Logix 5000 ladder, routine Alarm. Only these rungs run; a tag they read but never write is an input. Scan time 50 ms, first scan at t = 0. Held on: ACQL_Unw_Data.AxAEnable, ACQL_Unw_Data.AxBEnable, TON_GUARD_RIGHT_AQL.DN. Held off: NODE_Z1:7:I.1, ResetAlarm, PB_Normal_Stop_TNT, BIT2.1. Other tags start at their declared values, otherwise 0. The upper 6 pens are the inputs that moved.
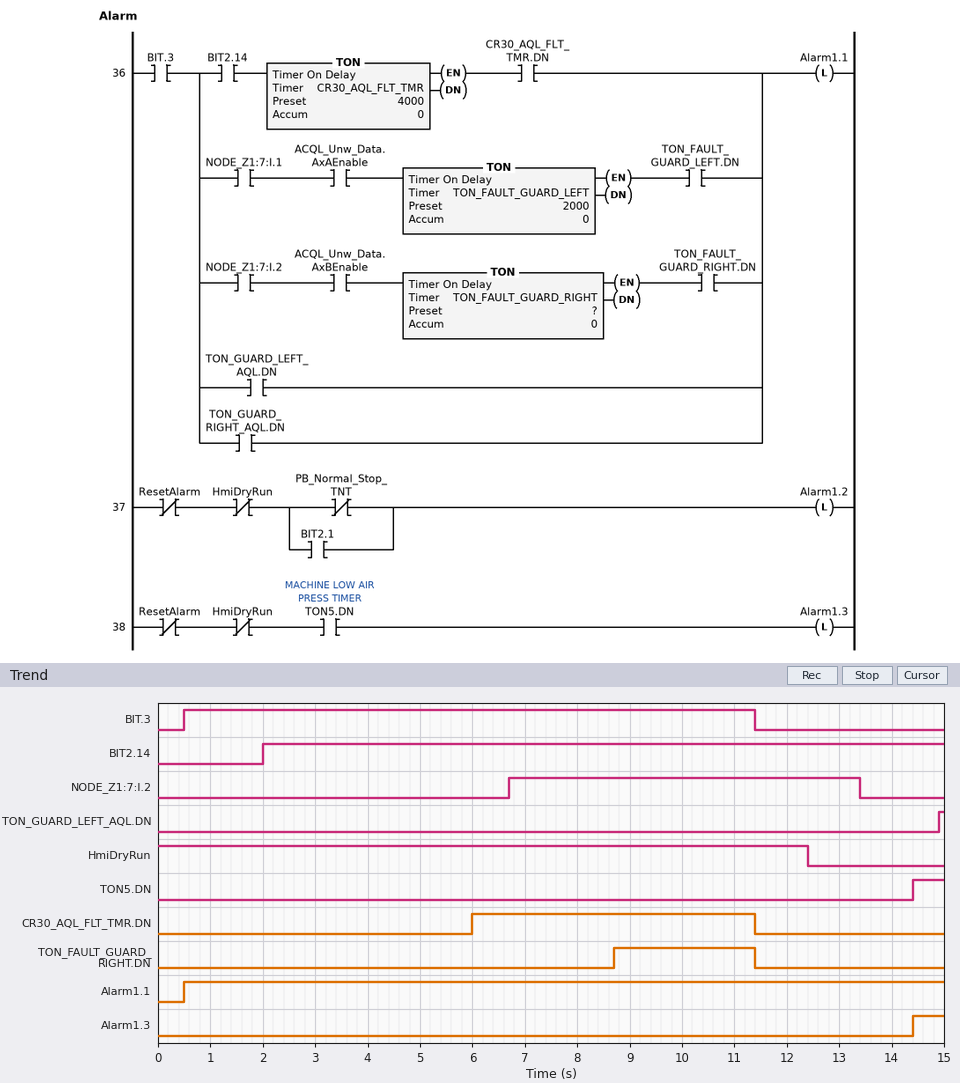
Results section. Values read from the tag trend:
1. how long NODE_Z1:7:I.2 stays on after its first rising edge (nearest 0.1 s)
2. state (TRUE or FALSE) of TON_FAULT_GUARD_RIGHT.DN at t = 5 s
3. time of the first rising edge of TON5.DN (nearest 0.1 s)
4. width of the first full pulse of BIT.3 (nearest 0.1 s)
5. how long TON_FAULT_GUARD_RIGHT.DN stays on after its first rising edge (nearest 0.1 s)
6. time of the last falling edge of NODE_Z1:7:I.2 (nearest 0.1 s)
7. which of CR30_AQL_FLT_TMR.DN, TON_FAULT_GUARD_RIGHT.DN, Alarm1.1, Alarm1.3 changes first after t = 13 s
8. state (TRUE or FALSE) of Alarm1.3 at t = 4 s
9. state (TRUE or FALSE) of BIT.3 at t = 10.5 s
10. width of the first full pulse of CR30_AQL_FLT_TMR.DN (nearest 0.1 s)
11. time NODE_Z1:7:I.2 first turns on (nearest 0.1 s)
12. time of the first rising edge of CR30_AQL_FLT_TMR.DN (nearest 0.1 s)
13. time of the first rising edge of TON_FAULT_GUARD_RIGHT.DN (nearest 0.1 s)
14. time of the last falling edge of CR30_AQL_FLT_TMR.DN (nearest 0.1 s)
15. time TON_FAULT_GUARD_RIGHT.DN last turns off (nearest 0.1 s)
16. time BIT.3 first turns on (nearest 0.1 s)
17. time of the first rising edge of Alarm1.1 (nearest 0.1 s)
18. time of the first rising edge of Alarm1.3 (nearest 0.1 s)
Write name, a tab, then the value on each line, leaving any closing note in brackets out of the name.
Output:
how long NODE_Z1:7:I.2 stays on after its first rising edge	6.7 s
state (TRUE or FALSE) of TON_FAULT_GUARD_RIGHT.DN at t = 5 s	FALSE
time of the first rising edge of TON5.DN	14.4 s
width of the first full pulse of BIT.3	10.9 s
how long TON_FAULT_GUARD_RIGHT.DN stays on after its first rising edge	2.7 s
time of the last falling edge of NODE_Z1:7:I.2	13.4 s
which of CR30_AQL_FLT_TMR.DN, TON_FAULT_GUARD_RIGHT.DN, Alarm1.1, Alarm1.3 changes first after t = 13 s	Alarm1.3
state (TRUE or FALSE) of Alarm1.3 at t = 4 s	FALSE
state (TRUE or FALSE) of BIT.3 at t = 10.5 s	TRUE
width of the first full pulse of CR30_AQL_FLT_TMR.DN	5.4 s
time NODE_Z1:7:I.2 first turns on	6.7 s
time of the first rising edge of CR30_AQL_FLT_TMR.DN	6.0 s
time of the first rising edge of TON_FAULT_GUARD_RIGHT.DN	8.7 s
time of the last falling edge of CR30_AQL_FLT_TMR.DN	11.4 s
time TON_FAULT_GUARD_RIGHT.DN last turns off	11.4 s
time BIT.3 first turns on	0.5 s
time of the first rising edge of Alarm1.1	0.5 s
time of the first rising edge of Alarm1.3	14.4 s
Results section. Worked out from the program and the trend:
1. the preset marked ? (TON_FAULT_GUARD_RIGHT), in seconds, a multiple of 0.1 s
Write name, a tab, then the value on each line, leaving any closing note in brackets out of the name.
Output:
the preset marked ? (TON_FAULT_GUARD_RIGHT), in seconds, a multiple of 0.1 s	2.0 s
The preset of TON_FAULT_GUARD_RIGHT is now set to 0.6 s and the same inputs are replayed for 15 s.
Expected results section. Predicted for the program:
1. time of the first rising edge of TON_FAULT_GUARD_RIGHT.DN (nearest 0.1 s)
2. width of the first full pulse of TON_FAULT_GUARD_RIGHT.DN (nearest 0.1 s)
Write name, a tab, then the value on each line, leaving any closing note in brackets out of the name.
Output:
time of the first rising edge of TON_FAULT_GUARD_RIGHT.DN	7.3 s
width of the first full pulse of TON_FAULT_GUARD_RIGHT.DN	4.1 s
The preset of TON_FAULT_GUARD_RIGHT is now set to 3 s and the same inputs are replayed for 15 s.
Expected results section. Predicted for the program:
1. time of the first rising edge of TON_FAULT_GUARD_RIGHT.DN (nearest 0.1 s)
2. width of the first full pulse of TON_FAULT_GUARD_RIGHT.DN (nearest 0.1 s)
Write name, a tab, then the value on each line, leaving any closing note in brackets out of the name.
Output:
time of the first rising edge of TON_FAULT_GUARD_RIGHT.DN	9.7 s
width of the first full pulse of TON_FAULT_GUARD_RIGHT.DN	1.7 s
